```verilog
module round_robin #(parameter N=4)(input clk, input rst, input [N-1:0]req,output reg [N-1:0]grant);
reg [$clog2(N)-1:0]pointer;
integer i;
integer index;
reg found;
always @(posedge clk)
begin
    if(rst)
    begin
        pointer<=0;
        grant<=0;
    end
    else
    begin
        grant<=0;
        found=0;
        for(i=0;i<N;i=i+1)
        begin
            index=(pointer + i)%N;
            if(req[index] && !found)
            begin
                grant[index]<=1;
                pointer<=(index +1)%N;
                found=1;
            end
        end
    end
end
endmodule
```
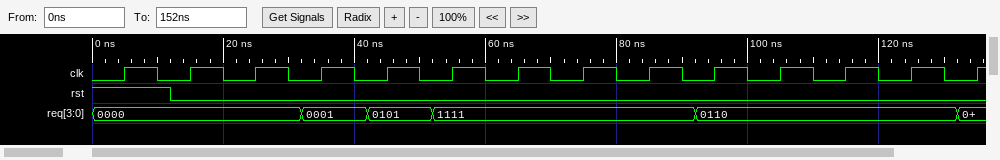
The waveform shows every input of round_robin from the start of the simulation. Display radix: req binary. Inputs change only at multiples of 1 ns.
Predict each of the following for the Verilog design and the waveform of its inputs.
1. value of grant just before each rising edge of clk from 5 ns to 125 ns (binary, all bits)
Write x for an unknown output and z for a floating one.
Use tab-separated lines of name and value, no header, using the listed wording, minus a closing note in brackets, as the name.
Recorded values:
value of grant just before each rising edge of clk from 5 ns to 125 ns	x, 0000, 0000, 0000, 0001, 0100, 1000, 0001, 0010, 0100, 0010, 0100, 0010
